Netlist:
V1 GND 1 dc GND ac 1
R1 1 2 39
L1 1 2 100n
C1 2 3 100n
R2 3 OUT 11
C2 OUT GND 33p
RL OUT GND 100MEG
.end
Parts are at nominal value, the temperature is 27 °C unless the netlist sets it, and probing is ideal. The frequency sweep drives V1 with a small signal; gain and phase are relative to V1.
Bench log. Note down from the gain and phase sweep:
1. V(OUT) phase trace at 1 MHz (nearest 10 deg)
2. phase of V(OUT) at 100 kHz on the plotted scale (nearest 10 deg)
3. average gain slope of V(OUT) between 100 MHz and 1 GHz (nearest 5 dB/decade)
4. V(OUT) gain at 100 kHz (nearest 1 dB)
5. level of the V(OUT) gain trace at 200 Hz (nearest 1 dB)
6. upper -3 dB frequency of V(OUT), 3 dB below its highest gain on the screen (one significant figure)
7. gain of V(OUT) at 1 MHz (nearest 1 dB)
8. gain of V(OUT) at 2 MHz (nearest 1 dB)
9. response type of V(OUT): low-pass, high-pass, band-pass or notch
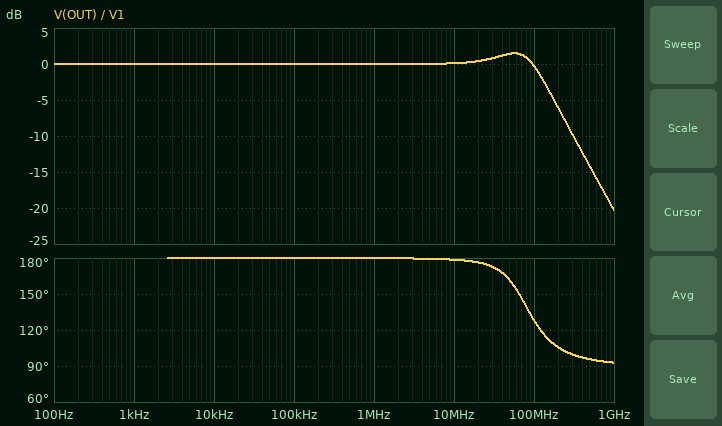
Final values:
180 deg
180 deg
-20 dB/decade
0 dB
0 dB
100 MHz
0 dB
0 dB
low-pass
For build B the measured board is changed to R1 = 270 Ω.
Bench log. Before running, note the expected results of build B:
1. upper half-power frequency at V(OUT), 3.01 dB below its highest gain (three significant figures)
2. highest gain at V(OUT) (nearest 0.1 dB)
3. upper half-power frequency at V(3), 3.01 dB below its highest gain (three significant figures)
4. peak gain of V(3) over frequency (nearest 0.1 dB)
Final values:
98.5 MHz
8.4 dB
98.7 MHz
8.5 dB
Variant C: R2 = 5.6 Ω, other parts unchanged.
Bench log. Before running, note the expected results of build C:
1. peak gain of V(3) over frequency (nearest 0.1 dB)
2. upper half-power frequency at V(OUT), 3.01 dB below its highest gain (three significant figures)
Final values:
1.8 dB
128 MHz
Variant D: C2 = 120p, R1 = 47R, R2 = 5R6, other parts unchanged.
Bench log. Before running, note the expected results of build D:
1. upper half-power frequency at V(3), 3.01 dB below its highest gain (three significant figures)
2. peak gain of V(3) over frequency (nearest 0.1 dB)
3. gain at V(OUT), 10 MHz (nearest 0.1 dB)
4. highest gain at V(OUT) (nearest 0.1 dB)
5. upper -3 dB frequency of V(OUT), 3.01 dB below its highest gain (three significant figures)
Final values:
54.6 MHz
4.1 dB
0.4 dB
4.0 dB
54.2 MHz
